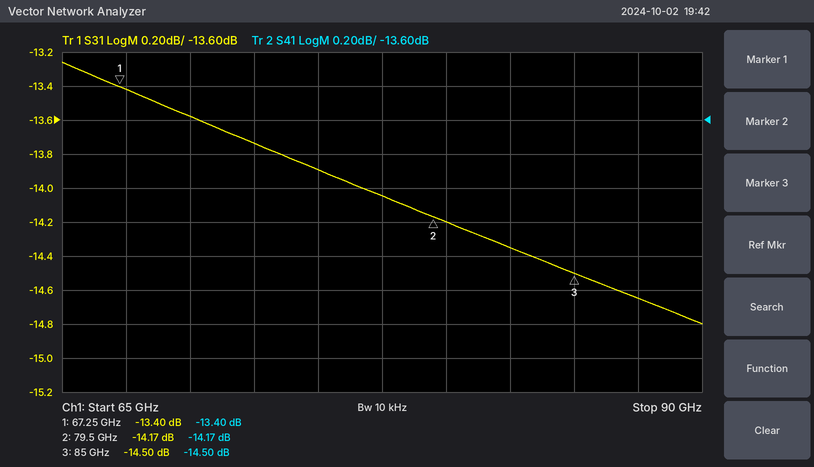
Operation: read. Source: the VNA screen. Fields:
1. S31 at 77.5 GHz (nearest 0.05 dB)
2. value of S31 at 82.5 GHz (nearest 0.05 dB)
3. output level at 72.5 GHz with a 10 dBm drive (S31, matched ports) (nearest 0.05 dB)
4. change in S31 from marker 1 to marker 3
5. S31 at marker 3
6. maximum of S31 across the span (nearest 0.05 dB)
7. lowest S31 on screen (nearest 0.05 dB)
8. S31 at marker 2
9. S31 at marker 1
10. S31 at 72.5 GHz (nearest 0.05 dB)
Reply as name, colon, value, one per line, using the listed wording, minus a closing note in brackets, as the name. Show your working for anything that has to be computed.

S31 at 77.5 GHz: -14.05 dB
value of S31 at 82.5 GHz: -14.35 dB
output level at 72.5 GHz with a 10 dBm drive (S31, matched ports): 10 dBm + (-13.75 dB) = -3.75 dBm
change in S31 from marker 1 to marker 3: -14.5 − (-13.4) = -1.10 dB
S31 at marker 3: -14.50 dB
maximum of S31 across the span: -13.25 dB
lowest S31 on screen: -14.80 dB
S31 at marker 2: -14.17 dB
S31 at marker 1: -13.40 dB
S31 at 72.5 GHz: -13.75 dB
